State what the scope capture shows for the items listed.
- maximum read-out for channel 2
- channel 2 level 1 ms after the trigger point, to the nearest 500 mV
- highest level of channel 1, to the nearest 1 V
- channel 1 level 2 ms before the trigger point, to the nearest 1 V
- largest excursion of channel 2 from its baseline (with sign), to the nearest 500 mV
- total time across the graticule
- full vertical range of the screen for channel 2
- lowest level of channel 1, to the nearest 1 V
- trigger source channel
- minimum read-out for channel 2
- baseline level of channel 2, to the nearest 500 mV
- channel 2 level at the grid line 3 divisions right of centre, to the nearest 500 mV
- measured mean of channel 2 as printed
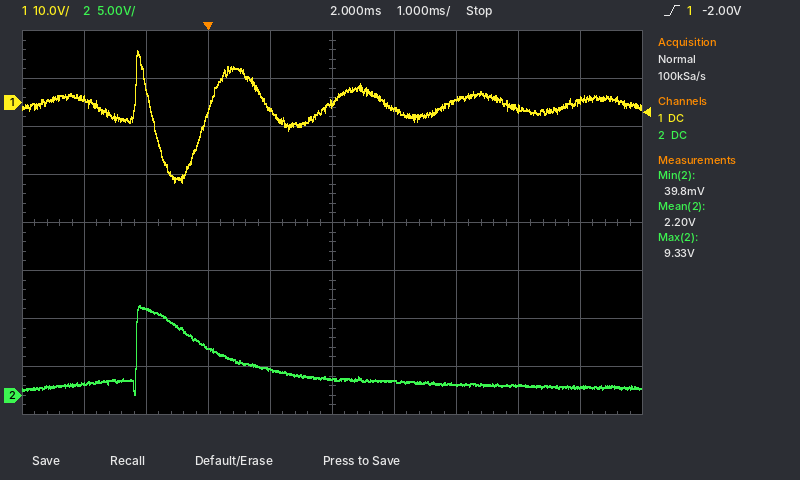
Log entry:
9.33 V
2.5 V
11 V
1 V
+8.0 V
10 ms
40 V
-17 V
channel 1
39.8 mV
1.0 V
1.0 V
2.20 V
